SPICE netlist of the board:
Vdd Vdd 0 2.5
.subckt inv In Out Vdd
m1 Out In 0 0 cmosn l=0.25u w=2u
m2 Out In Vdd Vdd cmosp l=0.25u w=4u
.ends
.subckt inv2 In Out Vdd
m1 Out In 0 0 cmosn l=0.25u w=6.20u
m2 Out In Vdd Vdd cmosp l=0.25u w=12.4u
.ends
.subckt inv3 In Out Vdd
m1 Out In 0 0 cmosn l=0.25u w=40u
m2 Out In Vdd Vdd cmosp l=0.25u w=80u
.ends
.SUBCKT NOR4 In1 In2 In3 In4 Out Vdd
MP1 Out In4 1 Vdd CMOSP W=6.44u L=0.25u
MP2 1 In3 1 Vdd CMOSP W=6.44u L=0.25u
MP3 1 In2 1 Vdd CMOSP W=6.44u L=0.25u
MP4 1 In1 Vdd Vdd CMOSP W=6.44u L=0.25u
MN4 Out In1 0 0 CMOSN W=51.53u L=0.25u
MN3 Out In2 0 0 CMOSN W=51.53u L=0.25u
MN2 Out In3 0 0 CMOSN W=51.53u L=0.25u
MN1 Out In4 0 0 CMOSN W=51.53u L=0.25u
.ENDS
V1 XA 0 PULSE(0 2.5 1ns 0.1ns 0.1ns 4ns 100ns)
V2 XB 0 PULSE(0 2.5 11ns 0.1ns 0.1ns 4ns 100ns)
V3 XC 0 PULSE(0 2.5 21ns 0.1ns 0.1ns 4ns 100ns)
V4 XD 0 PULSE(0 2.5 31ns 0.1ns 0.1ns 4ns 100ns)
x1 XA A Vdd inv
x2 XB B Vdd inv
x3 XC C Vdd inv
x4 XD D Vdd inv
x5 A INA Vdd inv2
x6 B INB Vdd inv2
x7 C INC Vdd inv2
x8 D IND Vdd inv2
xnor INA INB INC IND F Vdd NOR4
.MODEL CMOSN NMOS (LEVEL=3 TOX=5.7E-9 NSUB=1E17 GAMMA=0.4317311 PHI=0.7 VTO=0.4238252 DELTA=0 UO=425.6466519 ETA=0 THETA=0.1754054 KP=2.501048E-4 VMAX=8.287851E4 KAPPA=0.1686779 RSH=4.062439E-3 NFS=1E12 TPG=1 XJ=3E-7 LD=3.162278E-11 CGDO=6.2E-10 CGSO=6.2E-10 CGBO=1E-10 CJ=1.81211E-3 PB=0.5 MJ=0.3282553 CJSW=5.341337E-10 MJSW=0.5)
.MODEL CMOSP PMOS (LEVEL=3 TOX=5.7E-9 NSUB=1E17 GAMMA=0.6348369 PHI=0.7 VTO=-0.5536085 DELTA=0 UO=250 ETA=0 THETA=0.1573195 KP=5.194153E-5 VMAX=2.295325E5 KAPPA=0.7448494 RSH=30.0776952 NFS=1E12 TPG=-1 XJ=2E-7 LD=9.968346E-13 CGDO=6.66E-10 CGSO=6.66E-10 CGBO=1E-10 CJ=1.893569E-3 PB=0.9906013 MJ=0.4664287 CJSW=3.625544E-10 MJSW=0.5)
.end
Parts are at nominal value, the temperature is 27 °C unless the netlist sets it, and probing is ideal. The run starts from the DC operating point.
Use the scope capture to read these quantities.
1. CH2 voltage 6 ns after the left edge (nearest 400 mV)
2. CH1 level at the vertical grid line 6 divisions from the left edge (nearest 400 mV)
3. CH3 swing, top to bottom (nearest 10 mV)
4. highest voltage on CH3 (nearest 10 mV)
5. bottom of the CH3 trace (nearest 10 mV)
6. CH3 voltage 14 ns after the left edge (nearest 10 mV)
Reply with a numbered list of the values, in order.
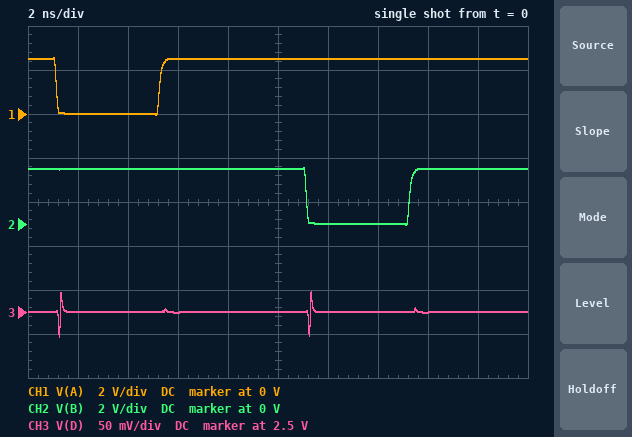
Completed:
1. 2.4 V
2. 2.4 V
3. 50 mV
4. 2.52 V
5. 2.47 V
6. 2.50 V
